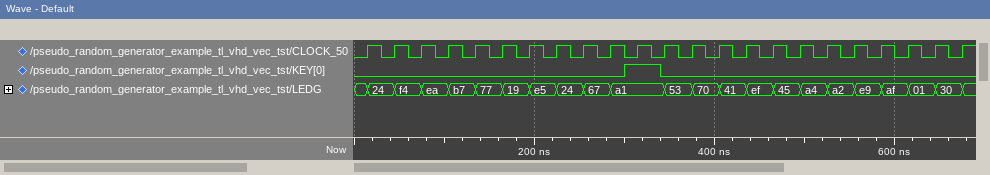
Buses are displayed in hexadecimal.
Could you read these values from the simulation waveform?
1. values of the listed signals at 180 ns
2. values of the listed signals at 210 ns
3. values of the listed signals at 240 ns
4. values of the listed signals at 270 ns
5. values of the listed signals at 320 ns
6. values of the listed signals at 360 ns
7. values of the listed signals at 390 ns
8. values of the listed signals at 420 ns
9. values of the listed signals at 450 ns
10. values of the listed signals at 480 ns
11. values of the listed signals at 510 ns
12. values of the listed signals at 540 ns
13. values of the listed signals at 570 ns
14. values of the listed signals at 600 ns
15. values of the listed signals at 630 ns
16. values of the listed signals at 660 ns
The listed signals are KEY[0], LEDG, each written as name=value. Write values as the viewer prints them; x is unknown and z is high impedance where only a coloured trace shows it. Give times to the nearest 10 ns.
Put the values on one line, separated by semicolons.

KEY[0]=0, LEDG=19; KEY[0]=0, LEDG=e5; KEY[0]=0, LEDG=24; KEY[0]=0, LEDG=67; KEY[0]=1, LEDG=a1; KEY[0]=0, LEDG=53; KEY[0]=0, LEDG=70; KEY[0]=0, LEDG=41; KEY[0]=0, LEDG=ef; KEY[0]=0, LEDG=45; KEY[0]=0, LEDG=a4; KEY[0]=0, LEDG=a2; KEY[0]=0, LEDG=e9; KEY[0]=0, LEDG=af; KEY[0]=0, LEDG=01; KEY[0]=0, LEDG=30
